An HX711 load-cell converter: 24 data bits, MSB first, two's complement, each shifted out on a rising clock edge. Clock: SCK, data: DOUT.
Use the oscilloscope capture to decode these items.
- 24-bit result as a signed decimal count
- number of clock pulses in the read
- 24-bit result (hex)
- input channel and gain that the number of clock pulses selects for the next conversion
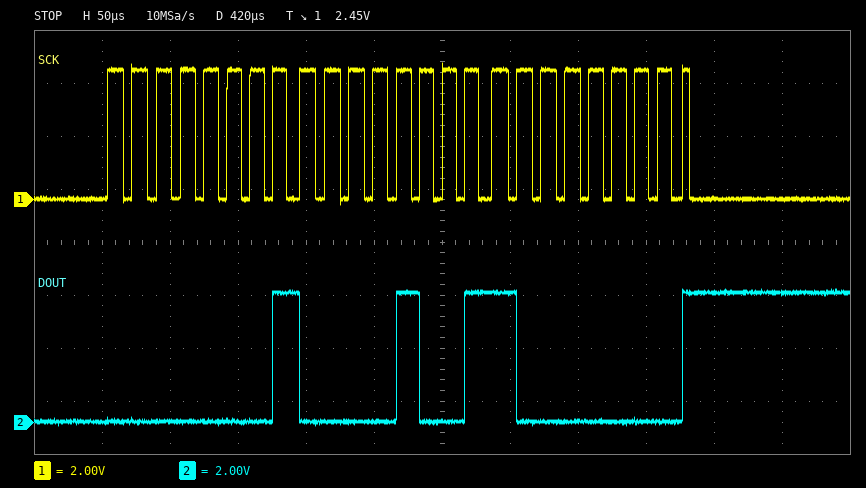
67968
25
0x010980
channel A, gain 128
